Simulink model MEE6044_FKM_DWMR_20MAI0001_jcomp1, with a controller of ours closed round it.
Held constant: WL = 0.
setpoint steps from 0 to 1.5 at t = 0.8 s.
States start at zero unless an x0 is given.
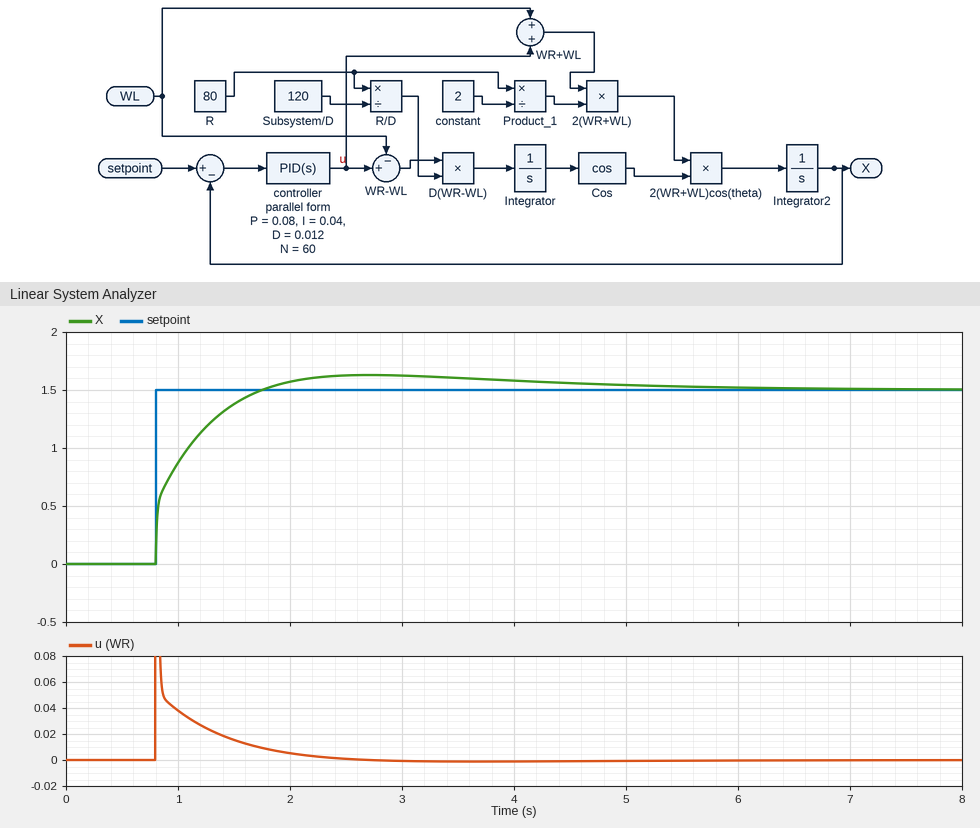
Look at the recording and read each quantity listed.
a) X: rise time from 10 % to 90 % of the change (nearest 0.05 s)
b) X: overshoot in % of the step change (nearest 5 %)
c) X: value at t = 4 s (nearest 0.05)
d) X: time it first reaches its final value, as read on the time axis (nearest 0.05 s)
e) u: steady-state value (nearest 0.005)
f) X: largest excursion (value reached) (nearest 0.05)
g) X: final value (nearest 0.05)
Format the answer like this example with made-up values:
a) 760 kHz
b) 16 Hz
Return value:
a) 0.65 s
b) 10 %
c) 1.60
d) 1.75 s
e) 0.000
f) 1.65
g) 1.50
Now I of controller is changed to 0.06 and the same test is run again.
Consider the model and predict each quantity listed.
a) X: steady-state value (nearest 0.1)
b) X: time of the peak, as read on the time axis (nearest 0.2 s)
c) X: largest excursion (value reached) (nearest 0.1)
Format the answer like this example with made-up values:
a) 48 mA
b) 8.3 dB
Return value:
a) 1.5
b) 2.4 s
c) 1.7
